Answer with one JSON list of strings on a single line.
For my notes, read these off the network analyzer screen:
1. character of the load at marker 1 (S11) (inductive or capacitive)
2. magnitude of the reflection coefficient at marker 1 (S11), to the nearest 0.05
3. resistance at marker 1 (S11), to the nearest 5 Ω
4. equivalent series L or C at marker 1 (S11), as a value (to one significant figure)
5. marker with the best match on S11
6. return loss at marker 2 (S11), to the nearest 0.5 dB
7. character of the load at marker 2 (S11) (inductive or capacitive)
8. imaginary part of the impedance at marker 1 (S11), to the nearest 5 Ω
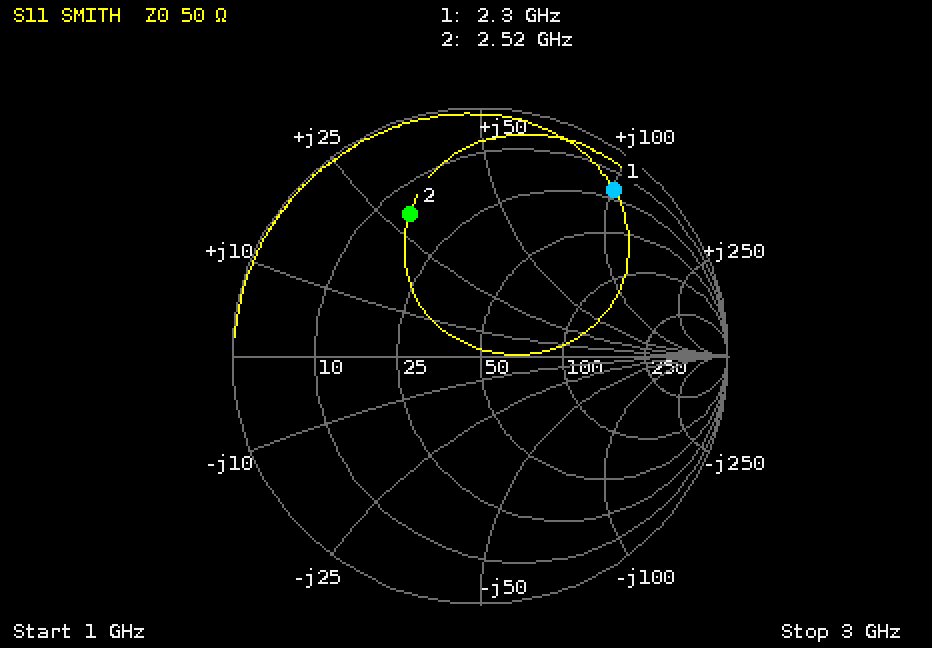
["inductive", "0.85", "20 Ω", "7 nH", "marker 2", "4.0 dB", "inductive", "+100 Ω"]
